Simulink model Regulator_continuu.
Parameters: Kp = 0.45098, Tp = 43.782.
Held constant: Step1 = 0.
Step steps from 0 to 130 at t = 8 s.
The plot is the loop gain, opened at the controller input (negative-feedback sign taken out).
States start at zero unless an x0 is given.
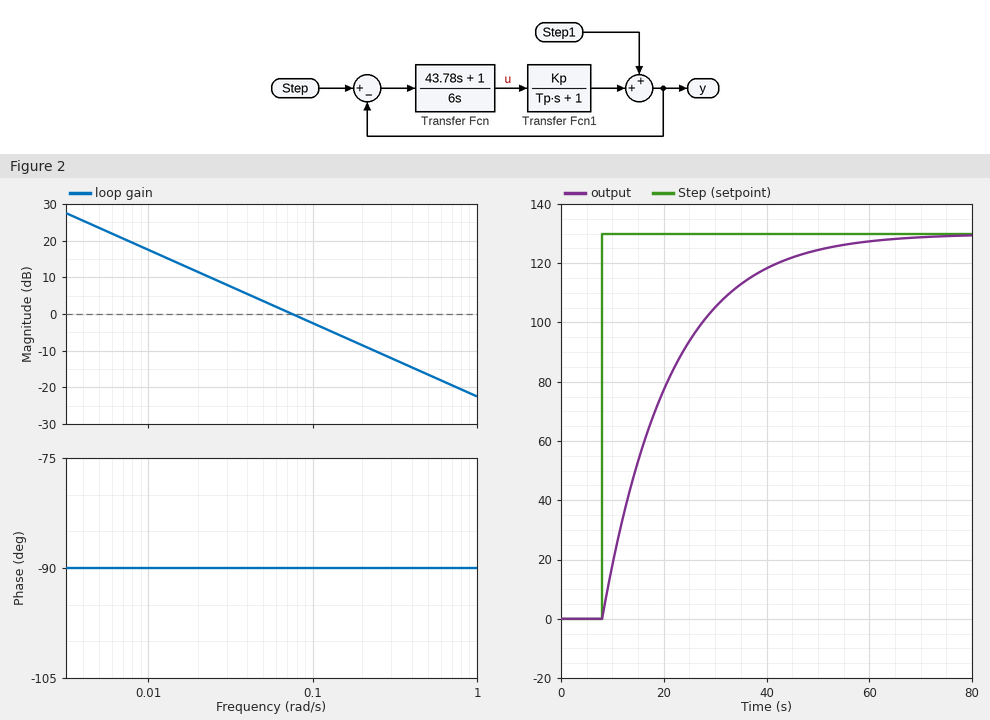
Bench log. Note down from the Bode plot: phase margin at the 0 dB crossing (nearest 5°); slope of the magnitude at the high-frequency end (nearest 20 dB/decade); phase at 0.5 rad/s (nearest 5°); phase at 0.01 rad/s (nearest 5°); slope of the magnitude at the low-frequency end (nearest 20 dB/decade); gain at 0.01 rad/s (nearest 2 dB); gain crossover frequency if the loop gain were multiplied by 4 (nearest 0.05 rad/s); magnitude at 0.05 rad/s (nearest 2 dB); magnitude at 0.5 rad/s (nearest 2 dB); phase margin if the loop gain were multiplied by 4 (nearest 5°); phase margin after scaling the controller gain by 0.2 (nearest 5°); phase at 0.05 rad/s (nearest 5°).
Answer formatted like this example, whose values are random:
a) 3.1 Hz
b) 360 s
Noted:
a) 90°
b) -20 dB/decade
c) -90°
d) -90°
e) -20 dB/decade
f) 18 dB
g) 0.30 rad/s
h) 4 dB
i) -16 dB
j) 90°
k) 90°
l) -90°
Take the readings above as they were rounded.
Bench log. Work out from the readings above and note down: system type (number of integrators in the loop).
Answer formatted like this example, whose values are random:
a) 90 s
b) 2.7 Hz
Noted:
a) 1
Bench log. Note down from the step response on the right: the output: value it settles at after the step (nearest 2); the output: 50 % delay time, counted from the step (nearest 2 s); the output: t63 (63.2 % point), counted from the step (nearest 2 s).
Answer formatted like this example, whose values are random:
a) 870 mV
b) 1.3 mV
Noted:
a) 130
b) 10 s
c) 14 s
